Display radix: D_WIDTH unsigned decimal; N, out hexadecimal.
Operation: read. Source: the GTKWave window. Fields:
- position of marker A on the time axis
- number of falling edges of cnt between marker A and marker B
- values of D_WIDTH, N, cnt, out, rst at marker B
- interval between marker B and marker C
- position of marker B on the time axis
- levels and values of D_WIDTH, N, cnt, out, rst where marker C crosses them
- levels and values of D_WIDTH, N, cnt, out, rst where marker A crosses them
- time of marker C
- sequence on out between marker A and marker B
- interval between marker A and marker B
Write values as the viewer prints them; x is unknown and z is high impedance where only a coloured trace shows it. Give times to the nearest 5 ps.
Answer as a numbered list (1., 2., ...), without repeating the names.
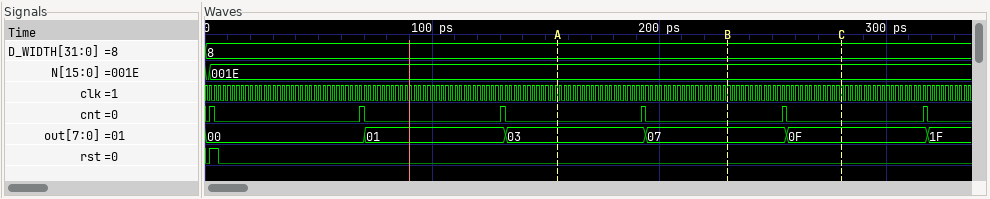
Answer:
1. 155 ps
2. 1
3. D_WIDTH=8, N=001E, cnt=0, out=07, rst=0
4. 50 ps
5. 230 ps
6. D_WIDTH=8, N=001E, cnt=0, out=0F, rst=0
7. D_WIDTH=8, N=001E, cnt=0, out=03, rst=0
8. 280 ps
9. 03, 07
10. 75 ps
